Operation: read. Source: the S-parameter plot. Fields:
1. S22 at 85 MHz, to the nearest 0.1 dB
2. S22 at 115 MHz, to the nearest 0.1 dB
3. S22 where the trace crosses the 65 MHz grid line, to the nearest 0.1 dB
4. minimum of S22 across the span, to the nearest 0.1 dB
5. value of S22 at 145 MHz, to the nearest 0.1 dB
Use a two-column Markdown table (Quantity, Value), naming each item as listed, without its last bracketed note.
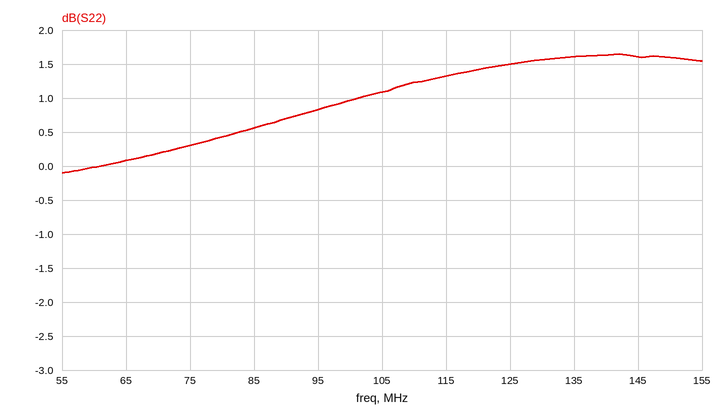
| Quantity | Value |
|---|---|
| S22 at 85 MHz, to the nearest 0.1 dB | 0.6 dB |
| S22 at 115 MHz, to the nearest 0.1 dB | 1.3 dB |
| S22 where the trace crosses the 65 MHz grid line, to the nearest 0.1 dB | 0.1 dB |
| minimum of S22 across the span, to the nearest 0.1 dB | -0.1 dB |
| value of S22 at 145 MHz, to the nearest 0.1 dB | 1.6 dB |
